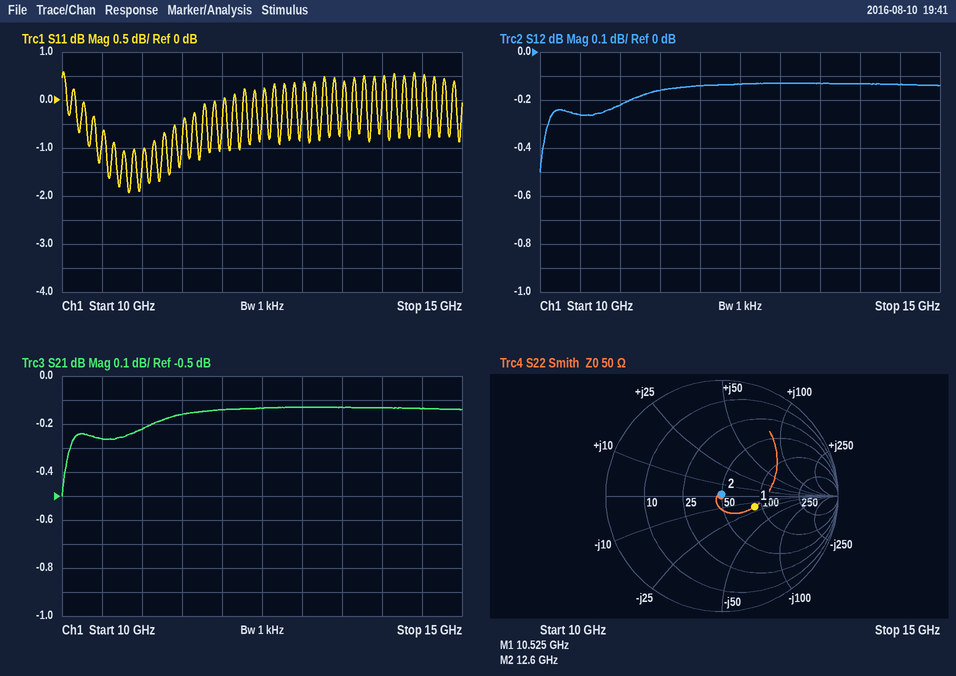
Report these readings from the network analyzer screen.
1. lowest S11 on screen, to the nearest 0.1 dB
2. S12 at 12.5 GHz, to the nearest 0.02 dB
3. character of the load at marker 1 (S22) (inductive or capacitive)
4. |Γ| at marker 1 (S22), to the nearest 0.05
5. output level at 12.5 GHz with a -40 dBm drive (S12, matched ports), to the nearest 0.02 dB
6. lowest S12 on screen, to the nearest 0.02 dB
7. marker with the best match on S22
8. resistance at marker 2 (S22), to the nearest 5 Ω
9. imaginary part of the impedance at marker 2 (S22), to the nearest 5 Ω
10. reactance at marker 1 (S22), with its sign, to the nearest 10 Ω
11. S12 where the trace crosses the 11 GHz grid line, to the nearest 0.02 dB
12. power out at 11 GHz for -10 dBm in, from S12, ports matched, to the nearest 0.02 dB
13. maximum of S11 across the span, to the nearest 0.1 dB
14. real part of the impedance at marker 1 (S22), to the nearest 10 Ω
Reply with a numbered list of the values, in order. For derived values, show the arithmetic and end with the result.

1. -1.9 dB
2. -0.14 dB
3. capacitive
4. 0.30
5. -40 dBm + (-0.14 dB) = -40.14 dBm
6. -0.50 dB
7. marker 2
8. 50 Ω
9. 0 Ω
10. -20 Ω
11. -0.22 dB
12. -10 dBm + (-0.22 dB) = -10.22 dBm
13. 0.6 dB
14. 90 Ω
